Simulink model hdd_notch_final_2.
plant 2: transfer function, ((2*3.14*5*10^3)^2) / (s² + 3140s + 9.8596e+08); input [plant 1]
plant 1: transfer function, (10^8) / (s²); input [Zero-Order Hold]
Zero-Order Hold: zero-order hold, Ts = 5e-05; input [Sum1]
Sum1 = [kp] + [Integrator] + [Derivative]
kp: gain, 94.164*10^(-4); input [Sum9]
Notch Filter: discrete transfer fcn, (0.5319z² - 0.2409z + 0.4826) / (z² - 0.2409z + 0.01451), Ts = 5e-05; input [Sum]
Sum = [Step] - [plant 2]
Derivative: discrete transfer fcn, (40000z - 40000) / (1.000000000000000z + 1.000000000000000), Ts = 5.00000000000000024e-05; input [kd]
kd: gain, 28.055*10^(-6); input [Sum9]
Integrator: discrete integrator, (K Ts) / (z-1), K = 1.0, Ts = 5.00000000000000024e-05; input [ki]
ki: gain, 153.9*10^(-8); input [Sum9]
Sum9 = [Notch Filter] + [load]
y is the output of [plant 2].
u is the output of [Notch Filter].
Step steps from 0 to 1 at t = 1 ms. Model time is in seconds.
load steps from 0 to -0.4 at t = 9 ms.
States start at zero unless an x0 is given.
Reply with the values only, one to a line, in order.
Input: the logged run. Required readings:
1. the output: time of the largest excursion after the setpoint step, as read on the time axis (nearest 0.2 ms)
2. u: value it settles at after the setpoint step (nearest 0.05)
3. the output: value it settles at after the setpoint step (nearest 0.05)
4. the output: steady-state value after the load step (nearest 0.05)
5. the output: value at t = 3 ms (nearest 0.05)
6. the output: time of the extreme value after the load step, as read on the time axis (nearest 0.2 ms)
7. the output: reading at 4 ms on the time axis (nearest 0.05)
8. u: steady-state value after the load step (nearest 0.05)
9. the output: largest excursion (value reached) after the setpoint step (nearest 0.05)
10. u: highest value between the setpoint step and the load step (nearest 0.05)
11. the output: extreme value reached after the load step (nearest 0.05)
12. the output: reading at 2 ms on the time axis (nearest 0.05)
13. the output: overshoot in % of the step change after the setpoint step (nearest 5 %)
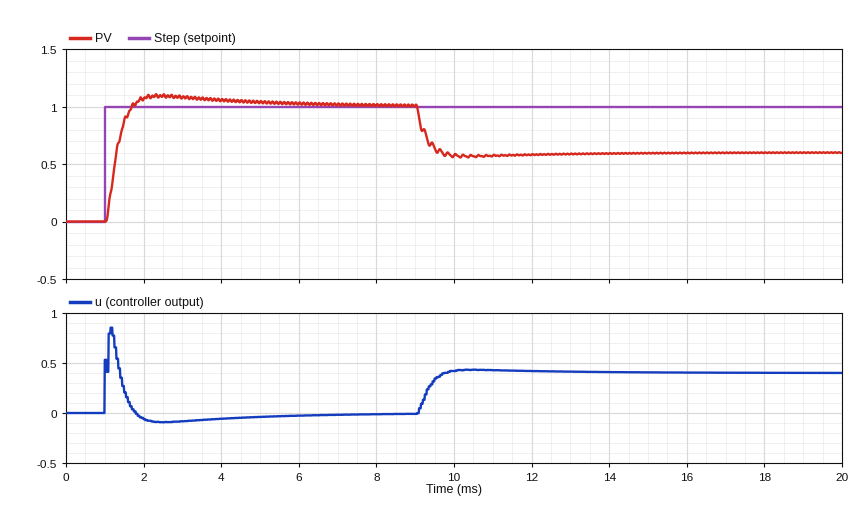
2.4 ms
0.00
1.00
0.60
1.10
10.2 ms
1.05
0.40
1.10
0.85
0.55
1.05
10 %
